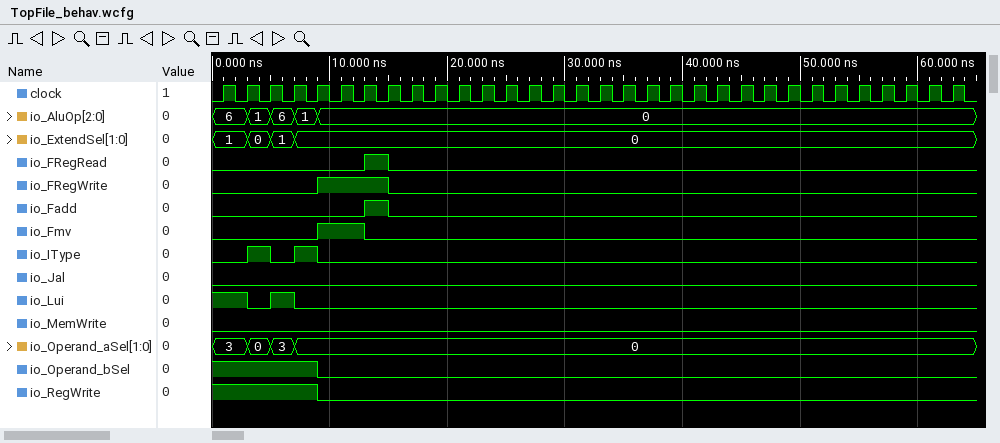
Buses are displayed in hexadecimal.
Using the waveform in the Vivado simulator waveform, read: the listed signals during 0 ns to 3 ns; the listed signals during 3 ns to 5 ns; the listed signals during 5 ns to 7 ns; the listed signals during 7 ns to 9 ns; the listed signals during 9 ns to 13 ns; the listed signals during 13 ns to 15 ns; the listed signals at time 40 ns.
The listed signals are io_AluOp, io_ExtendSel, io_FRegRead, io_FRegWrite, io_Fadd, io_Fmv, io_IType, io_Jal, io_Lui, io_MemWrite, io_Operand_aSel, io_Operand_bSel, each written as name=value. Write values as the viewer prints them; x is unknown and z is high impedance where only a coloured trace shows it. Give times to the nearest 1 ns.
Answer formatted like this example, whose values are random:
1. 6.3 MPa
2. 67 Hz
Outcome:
1. io_AluOp=6, io_ExtendSel=1, io_FRegRead=0, io_FRegWrite=0, io_Fadd=0, io_Fmv=0, io_IType=0, io_Jal=0, io_Lui=1, io_MemWrite=0, io_Operand_aSel=3, io_Operand_bSel=1
2. io_AluOp=1, io_ExtendSel=0, io_FRegRead=0, io_FRegWrite=0, io_Fadd=0, io_Fmv=0, io_IType=1, io_Jal=0, io_Lui=0, io_MemWrite=0, io_Operand_aSel=0, io_Operand_bSel=1
3. io_AluOp=6, io_ExtendSel=1, io_FRegRead=0, io_FRegWrite=0, io_Fadd=0, io_Fmv=0, io_IType=0, io_Jal=0, io_Lui=1, io_MemWrite=0, io_Operand_aSel=3, io_Operand_bSel=1
4. io_AluOp=1, io_ExtendSel=0, io_FRegRead=0, io_FRegWrite=0, io_Fadd=0, io_Fmv=0, io_IType=1, io_Jal=0, io_Lui=0, io_MemWrite=0, io_Operand_aSel=0, io_Operand_bSel=1
5. io_AluOp=0, io_ExtendSel=0, io_FRegRead=0, io_FRegWrite=1, io_Fadd=0, io_Fmv=1, io_IType=0, io_Jal=0, io_Lui=0, io_MemWrite=0, io_Operand_aSel=0, io_Operand_bSel=0
6. io_AluOp=0, io_ExtendSel=0, io_FRegRead=1, io_FRegWrite=1, io_Fadd=1, io_Fmv=0, io_IType=0, io_Jal=0, io_Lui=0, io_MemWrite=0, io_Operand_aSel=0, io_Operand_bSel=0
7. io_AluOp=0, io_ExtendSel=0, io_FRegRead=0, io_FRegWrite=0, io_Fadd=0, io_Fmv=0, io_IType=0, io_Jal=0, io_Lui=0, io_MemWrite=0, io_Operand_aSel=0, io_Operand_bSel=0
